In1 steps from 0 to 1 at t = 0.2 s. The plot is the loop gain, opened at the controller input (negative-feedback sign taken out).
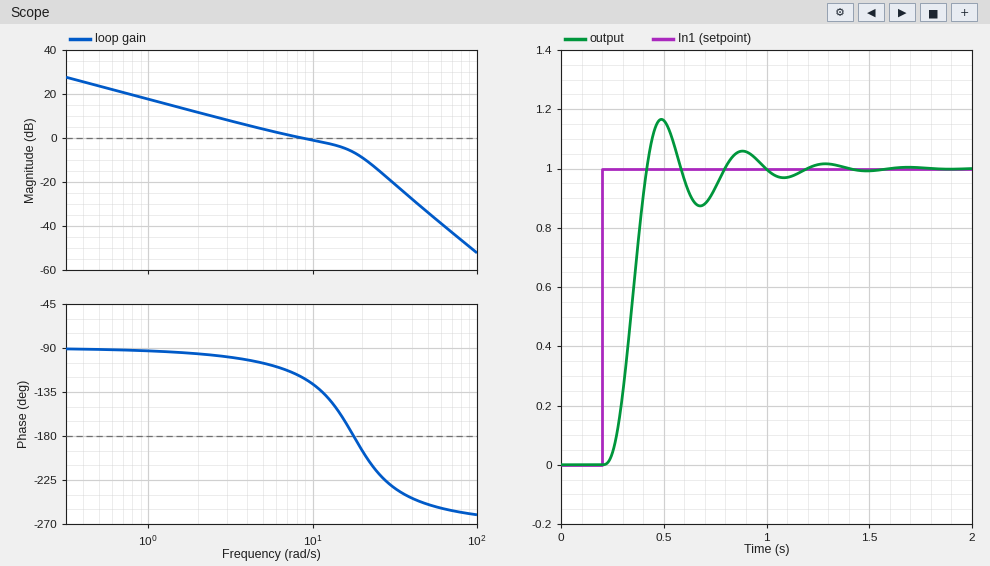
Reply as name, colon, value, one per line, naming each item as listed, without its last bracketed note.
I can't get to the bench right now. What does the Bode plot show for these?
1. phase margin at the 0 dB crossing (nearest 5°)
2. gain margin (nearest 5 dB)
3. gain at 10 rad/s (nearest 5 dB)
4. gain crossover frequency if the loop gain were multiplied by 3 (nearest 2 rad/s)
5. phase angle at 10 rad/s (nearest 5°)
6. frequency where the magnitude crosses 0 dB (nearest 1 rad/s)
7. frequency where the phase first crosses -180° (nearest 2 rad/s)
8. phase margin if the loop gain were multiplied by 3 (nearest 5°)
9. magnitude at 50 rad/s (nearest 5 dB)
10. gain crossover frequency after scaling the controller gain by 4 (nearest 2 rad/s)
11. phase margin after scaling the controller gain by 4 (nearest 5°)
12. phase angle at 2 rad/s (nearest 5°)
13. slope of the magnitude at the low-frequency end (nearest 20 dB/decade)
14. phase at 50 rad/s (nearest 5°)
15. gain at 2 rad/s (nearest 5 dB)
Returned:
phase margin at the 0 dB crossing: 60°
gain margin: 5 dB
gain at 10 rad/s: 0 dB
gain crossover frequency if the loop gain were multiplied by 3: 20 rad/s
phase angle at 10 rad/s: -125°
frequency where the magnitude crosses 0 dB: 9 rad/s
frequency where the phase first crosses -180°: 18 rad/s
phase margin if the loop gain were multiplied by 3: -20°
magnitude at 50 rad/s: -35 dB
gain crossover frequency after scaling the controller gain by 4: 22 rad/s
phase margin after scaling the controller gain by 4: -30°
phase angle at 2 rad/s: -95°
slope of the magnitude at the low-frequency end: -20 dB/decade
phase at 50 rad/s: -250°
gain at 2 rad/s: 10 dB
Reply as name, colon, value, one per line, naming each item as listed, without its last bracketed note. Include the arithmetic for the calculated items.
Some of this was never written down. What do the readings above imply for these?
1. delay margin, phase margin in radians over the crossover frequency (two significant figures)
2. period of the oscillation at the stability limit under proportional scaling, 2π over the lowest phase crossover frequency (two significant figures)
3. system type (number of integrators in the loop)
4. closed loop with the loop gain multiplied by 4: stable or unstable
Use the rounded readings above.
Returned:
delay margin, phase margin in radians over the crossover frequency: 60 × π / 180 / 9 = 0.12 s
period of the oscillation at the stability limit under proportional scaling, 2π over the lowest phase crossover frequency: 2π / 18 = 0.35 s
system type: 1
closed loop with the loop gain multiplied by 4: stable or unstable: unstable
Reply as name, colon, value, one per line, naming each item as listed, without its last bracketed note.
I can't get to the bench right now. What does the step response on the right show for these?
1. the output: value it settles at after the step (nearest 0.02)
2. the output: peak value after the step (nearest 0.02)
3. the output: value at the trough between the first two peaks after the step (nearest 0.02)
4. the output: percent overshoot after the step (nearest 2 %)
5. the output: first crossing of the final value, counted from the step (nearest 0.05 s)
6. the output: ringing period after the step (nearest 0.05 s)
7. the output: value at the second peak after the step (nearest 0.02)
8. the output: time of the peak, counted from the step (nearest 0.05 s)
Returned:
the output: value it settles at after the step: 1.00
the output: peak value after the step: 1.16
the output: value at the trough between the first two peaks after the step: 0.88
the output: percent overshoot after the step: 16 %
the output: first crossing of the final value, counted from the step: 0.20 s
the output: ringing period after the step: 0.40 s
the output: value at the second peak after the step: 1.06
the output: time of the peak, counted from the step: 0.30 s
